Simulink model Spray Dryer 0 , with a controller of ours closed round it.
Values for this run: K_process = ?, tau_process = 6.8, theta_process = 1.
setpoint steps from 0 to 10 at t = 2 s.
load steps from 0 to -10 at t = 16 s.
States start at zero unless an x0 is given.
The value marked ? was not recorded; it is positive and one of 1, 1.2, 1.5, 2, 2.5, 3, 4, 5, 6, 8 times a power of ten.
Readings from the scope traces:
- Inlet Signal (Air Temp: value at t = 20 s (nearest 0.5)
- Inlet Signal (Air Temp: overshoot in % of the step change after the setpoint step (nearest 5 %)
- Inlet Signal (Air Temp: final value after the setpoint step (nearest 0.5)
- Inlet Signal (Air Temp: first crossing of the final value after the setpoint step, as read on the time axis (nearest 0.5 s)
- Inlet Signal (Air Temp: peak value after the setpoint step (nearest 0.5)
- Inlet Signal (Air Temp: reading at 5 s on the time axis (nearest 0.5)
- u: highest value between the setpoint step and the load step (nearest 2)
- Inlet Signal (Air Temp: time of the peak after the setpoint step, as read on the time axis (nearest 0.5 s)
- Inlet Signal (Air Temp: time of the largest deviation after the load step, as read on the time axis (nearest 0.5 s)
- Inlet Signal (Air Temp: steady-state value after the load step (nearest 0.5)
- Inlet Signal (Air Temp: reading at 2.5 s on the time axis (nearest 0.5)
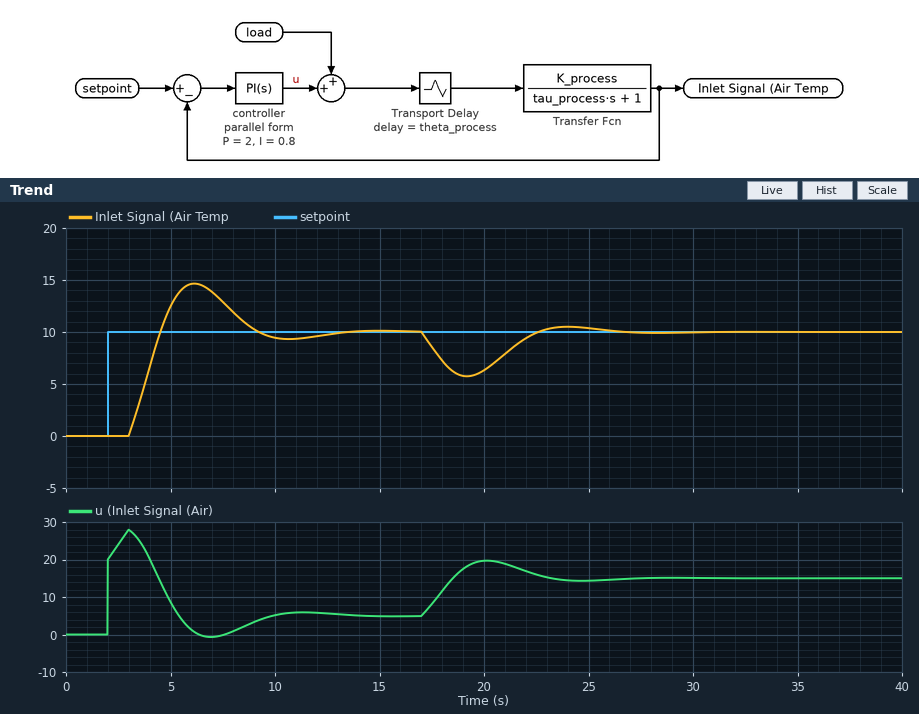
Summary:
6.5
45 %
10.0
4.5 s
14.5
12.5
28
6.0 s
19.0 s
10.0
0.0
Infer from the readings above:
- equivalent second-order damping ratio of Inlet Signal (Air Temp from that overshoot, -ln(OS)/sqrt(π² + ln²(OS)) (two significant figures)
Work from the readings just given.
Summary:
0.25
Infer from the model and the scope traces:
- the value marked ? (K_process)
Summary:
2
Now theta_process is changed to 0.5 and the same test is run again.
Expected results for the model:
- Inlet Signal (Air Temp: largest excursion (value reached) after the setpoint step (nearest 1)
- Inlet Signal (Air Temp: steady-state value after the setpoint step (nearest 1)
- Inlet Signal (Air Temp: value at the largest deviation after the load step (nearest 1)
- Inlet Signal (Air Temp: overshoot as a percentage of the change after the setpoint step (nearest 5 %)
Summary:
12
10
7
20 %
